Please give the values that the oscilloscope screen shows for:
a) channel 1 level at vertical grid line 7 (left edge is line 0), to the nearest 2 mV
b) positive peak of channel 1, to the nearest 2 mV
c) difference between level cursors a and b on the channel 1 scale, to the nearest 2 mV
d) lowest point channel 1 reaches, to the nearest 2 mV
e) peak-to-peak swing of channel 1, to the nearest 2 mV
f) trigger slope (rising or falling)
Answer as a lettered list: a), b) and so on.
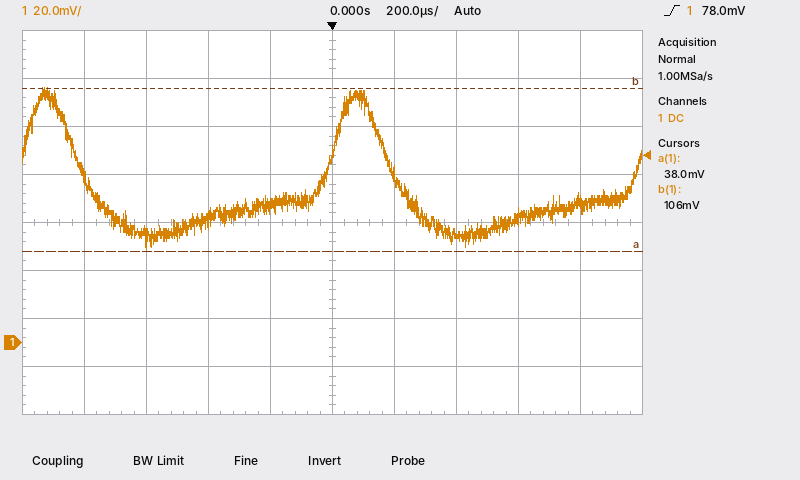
a) 46 mV
b) 106 mV
c) 68 mV
d) 38 mV
e) 68 mV
f) rising
